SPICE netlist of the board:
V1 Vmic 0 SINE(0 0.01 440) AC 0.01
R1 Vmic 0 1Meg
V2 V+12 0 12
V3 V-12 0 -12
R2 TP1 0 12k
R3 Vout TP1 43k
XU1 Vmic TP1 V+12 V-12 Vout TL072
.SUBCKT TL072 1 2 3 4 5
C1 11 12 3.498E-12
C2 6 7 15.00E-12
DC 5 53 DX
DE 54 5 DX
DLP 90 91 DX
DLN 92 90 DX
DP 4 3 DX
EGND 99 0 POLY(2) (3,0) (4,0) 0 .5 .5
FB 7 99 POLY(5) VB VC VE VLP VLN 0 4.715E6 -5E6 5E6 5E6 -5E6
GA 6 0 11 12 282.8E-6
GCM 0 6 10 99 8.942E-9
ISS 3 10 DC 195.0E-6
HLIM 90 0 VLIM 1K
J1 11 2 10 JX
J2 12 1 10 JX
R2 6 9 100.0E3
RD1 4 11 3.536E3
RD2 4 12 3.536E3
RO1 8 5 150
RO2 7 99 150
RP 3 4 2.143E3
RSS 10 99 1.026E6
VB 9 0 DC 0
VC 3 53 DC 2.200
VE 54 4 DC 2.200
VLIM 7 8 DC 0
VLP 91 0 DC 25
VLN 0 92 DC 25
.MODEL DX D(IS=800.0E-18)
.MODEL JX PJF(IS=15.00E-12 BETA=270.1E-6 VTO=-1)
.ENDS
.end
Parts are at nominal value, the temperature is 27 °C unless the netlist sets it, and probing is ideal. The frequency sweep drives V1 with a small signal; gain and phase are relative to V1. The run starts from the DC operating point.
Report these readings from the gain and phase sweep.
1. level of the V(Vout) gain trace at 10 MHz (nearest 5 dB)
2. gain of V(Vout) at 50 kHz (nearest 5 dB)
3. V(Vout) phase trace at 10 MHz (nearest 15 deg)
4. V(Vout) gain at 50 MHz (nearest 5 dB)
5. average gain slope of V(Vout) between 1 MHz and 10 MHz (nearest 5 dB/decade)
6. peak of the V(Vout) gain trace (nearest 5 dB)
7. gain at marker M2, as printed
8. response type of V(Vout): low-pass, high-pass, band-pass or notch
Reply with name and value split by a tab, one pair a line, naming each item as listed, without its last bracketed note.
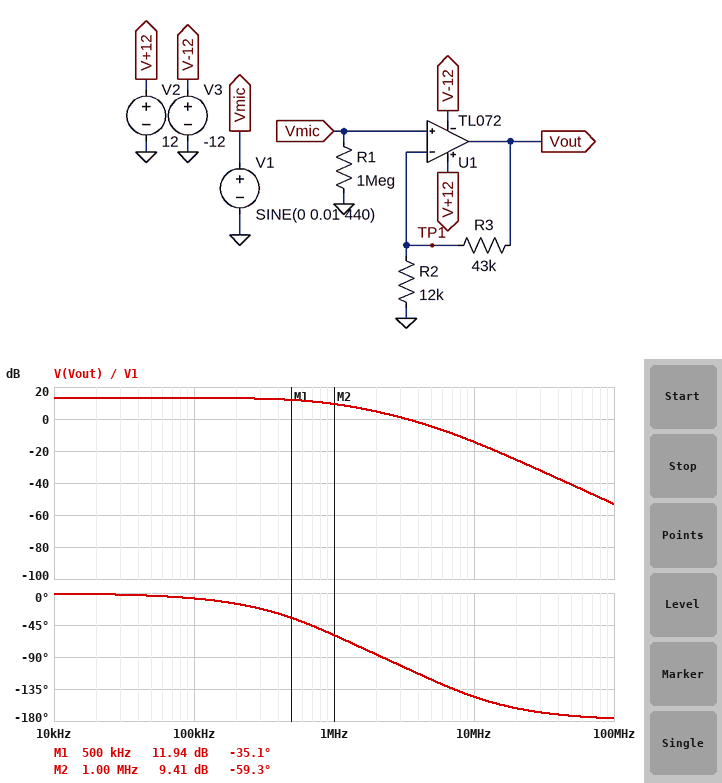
level of the V(Vout) gain trace at 10 MHz	-15 dB
gain of V(Vout) at 50 kHz	15 dB
V(Vout) phase trace at 10 MHz	-150 deg
V(Vout) gain at 50 MHz	-40 dB
average gain slope of V(Vout) between 1 MHz and 10 MHz	-25 dB/decade
peak of the V(Vout) gain trace	15 dB
gain at marker M2, as printed	9.41 dB
response type of V(Vout): low-pass, high-pass, band-pass or notch	low-pass
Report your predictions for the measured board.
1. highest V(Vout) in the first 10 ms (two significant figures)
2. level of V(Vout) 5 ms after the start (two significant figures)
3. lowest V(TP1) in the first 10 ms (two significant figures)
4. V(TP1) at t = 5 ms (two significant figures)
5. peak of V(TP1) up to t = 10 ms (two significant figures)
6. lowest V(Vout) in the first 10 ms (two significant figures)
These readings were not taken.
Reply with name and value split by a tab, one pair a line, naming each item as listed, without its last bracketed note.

highest V(Vout) in the first 10 ms	46 mV
level of V(Vout) 5 ms after the start	44 mV
lowest V(TP1) in the first 10 ms	-10 mV
V(TP1) at t = 5 ms	9.5 mV
peak of V(TP1) up to t = 10 ms	10 mV
lowest V(Vout) in the first 10 ms	-46 mV
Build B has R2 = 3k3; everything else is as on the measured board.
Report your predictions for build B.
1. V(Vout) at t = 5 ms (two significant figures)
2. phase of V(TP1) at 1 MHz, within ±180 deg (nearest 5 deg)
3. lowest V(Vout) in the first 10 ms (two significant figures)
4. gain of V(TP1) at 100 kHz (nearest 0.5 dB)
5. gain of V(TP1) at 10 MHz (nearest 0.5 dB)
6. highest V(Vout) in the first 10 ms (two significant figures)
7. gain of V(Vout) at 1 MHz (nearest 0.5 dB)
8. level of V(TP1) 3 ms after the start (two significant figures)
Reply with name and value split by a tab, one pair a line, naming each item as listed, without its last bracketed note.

V(Vout) at t = 5 ms	130 mV
phase of V(TP1) at 1 MHz, within ±180 deg	-85 deg
lowest V(Vout) in the first 10 ms	-140 mV
gain of V(TP1) at 100 kHz	-0.5 dB
gain of V(TP1) at 10 MHz	-37.5 dB
highest V(Vout) in the first 10 ms	140 mV
gain of V(Vout) at 1 MHz	10.5 dB
level of V(TP1) 3 ms after the start	9.1 mV
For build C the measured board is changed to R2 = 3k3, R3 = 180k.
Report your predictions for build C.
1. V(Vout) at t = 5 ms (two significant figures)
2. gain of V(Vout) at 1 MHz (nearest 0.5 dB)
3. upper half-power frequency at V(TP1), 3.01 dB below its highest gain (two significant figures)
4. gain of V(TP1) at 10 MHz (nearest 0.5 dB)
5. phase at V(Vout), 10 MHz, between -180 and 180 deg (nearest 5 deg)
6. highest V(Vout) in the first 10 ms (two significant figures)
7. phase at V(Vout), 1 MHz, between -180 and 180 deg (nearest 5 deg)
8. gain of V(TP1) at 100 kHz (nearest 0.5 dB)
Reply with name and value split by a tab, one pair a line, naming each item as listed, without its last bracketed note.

V(Vout) at t = 5 ms	530 mV
gain of V(Vout) at 1 MHz	10.5 dB
upper half-power frequency at V(TP1), 3.01 dB below its highest gain	63 kHz
gain of V(TP1) at 10 MHz	-49.5 dB
phase at V(Vout), 10 MHz, between -180 and 180 deg	-145 deg
highest V(Vout) in the first 10 ms	560 mV
phase at V(Vout), 1 MHz, between -180 and 180 deg	-95 deg
gain of V(TP1) at 100 kHz	-5.5 dB
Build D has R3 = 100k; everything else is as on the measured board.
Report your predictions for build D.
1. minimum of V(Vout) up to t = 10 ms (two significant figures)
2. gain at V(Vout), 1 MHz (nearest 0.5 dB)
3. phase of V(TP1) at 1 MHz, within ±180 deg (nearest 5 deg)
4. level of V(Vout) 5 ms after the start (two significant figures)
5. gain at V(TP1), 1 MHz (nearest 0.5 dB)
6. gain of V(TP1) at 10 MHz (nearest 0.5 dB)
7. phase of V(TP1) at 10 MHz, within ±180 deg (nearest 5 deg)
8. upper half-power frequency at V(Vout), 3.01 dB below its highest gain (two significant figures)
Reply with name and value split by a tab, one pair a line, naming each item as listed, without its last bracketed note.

minimum of V(Vout) up to t = 10 ms	-93 mV
gain at V(Vout), 1 MHz	10.5 dB
phase of V(TP1) at 1 MHz, within ±180 deg	-80 deg
level of V(Vout) 5 ms after the start	89 mV
gain at V(TP1), 1 MHz	-9.0 dB
gain of V(TP1) at 10 MHz	-34.0 dB
phase of V(TP1) at 10 MHz, within ±180 deg	-145 deg
upper half-power frequency at V(Vout), 3.01 dB below its highest gain	390 kHz
